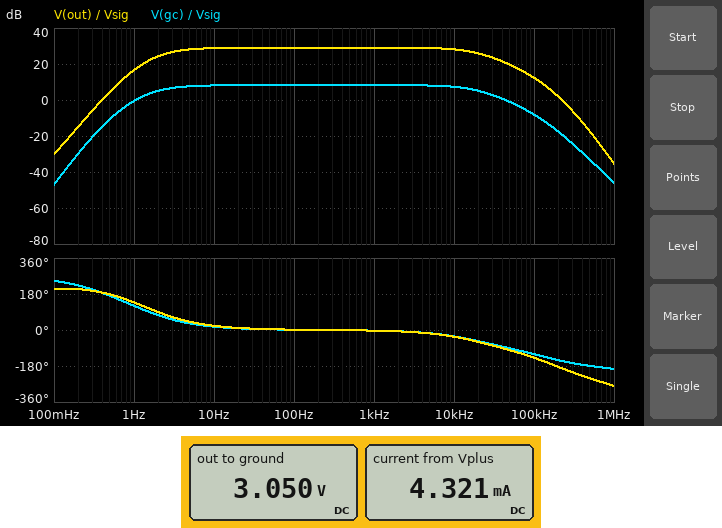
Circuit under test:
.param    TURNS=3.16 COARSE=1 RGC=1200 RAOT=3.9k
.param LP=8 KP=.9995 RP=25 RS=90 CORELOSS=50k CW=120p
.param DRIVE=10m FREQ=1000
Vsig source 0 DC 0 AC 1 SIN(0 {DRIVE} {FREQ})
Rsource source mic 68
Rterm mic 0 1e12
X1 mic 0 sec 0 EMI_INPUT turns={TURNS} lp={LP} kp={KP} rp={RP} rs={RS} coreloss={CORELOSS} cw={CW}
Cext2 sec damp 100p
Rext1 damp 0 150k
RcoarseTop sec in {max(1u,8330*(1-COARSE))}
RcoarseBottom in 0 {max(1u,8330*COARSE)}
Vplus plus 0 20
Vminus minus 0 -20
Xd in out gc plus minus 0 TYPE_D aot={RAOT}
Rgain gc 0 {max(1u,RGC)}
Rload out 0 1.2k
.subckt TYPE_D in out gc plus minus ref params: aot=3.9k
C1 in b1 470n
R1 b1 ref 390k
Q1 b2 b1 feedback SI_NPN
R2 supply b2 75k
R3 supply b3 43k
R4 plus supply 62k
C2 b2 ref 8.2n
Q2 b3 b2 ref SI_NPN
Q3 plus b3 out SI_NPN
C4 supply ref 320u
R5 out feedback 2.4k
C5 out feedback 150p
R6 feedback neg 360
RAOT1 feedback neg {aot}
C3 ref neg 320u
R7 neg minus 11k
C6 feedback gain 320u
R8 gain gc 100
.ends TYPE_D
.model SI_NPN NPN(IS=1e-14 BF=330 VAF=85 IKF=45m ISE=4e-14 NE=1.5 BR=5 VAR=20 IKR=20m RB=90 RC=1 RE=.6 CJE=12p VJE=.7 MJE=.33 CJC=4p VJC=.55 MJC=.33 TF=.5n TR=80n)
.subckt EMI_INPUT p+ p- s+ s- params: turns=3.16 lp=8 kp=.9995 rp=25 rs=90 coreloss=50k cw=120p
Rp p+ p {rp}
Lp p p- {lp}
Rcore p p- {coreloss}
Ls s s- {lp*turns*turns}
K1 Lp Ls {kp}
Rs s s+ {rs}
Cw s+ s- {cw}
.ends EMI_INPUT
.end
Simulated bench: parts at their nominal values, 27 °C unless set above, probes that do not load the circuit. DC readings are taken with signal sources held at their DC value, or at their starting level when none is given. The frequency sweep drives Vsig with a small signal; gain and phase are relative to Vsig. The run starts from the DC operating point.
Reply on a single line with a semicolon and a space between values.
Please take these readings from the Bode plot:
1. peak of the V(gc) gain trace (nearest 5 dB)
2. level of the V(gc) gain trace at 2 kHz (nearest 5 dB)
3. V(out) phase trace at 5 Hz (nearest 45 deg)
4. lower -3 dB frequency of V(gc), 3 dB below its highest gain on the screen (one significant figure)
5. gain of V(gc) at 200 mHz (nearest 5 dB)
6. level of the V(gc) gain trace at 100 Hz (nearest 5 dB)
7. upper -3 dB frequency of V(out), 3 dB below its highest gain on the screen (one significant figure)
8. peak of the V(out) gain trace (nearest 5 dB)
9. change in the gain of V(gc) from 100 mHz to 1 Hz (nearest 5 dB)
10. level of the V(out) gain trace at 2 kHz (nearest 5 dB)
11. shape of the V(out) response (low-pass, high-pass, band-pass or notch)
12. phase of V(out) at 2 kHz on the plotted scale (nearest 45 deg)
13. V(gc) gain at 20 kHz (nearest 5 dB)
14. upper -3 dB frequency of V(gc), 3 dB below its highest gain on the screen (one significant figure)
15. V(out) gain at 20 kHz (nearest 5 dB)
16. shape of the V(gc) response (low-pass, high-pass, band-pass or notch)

10 dB; 10 dB; 45 deg; 2 Hz; -30 dB; 10 dB; 20 kHz; 30 dB; 45 dB; 30 dB; band-pass; 0 deg; 5 dB; 20 kHz; 25 dB; band-pass
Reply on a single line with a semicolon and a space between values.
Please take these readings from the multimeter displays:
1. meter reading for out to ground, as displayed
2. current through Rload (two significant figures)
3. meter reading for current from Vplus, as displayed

3.050 V; 2.5 mA; 4.321 mA
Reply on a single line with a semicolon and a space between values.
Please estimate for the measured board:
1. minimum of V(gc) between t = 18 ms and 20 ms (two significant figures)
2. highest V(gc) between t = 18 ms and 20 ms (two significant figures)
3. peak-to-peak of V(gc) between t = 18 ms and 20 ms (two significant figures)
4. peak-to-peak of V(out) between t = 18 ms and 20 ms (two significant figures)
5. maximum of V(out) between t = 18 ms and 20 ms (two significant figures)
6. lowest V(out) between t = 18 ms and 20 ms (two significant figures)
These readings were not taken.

-26 mV; 26 mV; 52 mV; 570 mV; 3.3 V; 2.8 V
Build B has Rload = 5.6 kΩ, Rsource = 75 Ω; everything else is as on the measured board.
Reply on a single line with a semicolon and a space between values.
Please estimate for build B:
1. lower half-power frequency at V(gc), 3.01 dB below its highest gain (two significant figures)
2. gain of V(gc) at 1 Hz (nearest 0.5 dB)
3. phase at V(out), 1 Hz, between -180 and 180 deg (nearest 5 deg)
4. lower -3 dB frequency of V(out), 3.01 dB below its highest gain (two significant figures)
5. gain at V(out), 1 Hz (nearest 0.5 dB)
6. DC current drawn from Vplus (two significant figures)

2.2 Hz; -1.0 dB; 140 deg; 2.7 Hz; 16.0 dB; 2.3 mA
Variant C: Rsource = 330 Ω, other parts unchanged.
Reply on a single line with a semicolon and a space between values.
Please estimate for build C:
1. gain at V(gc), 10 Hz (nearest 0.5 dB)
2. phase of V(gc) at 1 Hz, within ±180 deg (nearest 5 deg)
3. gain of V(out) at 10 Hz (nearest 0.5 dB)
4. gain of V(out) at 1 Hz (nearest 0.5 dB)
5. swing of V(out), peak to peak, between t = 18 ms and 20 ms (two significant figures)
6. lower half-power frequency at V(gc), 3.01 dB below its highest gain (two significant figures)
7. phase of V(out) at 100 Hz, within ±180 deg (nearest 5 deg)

5.0 dB; 140 deg; 26.0 dB; 6.0 dB; 440 mV; 5.1 Hz; 5 deg
